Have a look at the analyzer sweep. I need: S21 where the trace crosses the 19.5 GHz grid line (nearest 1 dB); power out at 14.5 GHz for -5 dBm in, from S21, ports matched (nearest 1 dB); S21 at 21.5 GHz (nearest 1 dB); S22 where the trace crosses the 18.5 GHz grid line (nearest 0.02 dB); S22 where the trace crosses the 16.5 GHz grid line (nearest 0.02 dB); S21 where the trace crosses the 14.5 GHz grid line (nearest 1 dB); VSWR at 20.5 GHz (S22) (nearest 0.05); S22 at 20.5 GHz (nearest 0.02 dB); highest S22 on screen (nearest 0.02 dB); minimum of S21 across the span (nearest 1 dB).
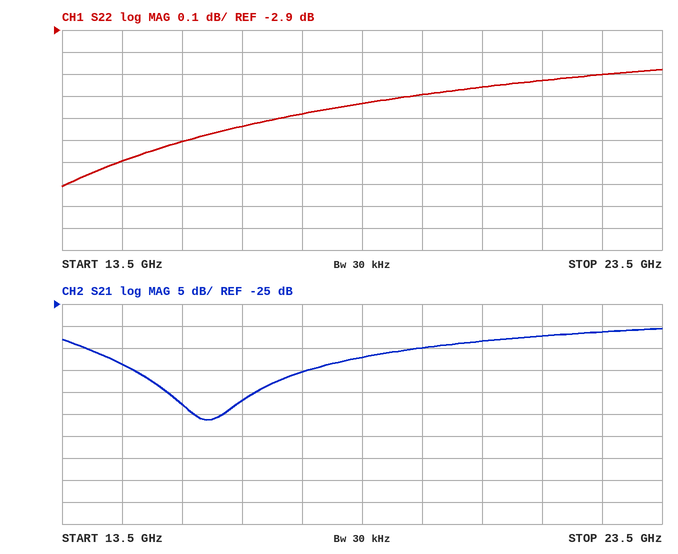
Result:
-35 dB
-44 dBm
-32 dB
-3.24 dB
-3.34 dB
-39 dB
5.55
-3.16 dB
-3.08 dB
-51 dB
